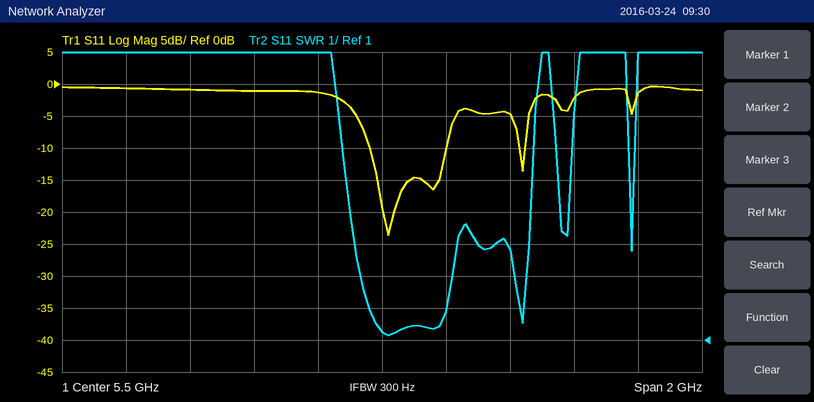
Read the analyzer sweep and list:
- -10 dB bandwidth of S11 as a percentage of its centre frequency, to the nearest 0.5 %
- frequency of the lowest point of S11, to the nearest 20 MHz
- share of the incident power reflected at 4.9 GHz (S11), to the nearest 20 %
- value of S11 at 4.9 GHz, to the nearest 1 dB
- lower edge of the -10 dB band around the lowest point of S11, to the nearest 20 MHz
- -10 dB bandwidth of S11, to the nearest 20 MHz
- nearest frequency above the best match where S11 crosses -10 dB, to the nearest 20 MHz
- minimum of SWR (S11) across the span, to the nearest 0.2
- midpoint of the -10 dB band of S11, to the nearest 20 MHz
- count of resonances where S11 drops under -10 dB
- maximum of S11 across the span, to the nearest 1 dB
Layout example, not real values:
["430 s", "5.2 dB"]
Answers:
["4.5 %", "5.52 GHz", "80 %", "-1 dB", "5.46 GHz", "240 MHz", "5.70 GHz", "1.2", "5.58 GHz", "2", "0 dB"]
